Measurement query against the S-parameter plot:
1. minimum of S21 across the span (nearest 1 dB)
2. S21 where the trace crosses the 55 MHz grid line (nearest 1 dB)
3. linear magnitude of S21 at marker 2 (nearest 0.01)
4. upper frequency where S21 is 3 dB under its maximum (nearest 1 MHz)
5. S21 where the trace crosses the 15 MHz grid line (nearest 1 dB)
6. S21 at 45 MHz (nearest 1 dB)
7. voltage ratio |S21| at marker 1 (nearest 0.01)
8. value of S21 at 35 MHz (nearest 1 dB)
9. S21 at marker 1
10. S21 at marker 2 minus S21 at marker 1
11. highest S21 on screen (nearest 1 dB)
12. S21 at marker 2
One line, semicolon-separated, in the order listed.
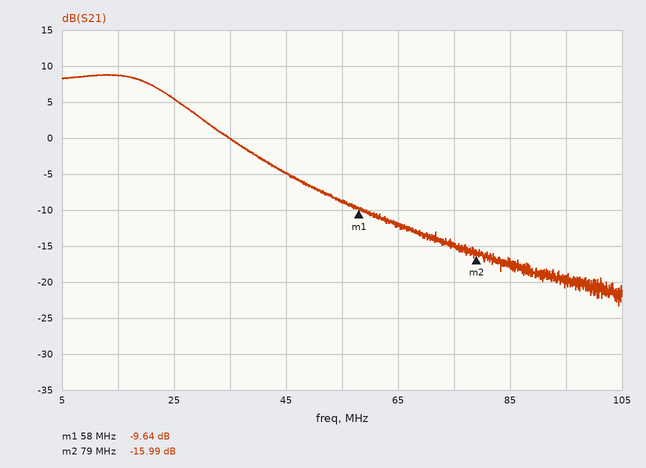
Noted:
-23 dB; -9 dB; 0.16; 24 MHz; 9 dB; -5 dB; 0.33; 0 dB; -9.64 dB; -6.35 dB; 9 dB; -15.99 dB
